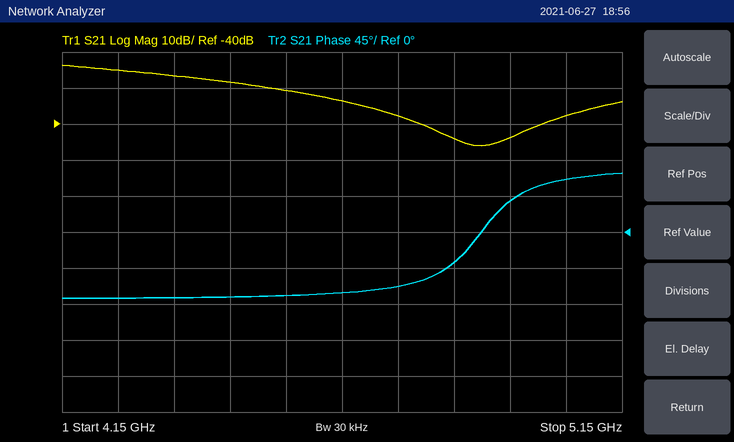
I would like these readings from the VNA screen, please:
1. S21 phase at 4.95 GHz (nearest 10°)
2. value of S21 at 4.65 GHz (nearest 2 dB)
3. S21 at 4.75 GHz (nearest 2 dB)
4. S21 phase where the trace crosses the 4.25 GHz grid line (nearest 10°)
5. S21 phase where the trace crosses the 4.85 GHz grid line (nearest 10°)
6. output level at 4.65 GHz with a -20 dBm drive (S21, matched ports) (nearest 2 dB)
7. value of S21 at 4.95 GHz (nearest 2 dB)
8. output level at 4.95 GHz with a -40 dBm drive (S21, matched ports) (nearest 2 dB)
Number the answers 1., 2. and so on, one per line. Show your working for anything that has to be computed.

1. 40°
2. -34 dB
3. -38 dB
4. -80°
5. -40°
6. -20 dBm + (-34 dB) = -54 dBm
7. -44 dB
8. -40 dBm + (-44 dB) = -84 dBm
